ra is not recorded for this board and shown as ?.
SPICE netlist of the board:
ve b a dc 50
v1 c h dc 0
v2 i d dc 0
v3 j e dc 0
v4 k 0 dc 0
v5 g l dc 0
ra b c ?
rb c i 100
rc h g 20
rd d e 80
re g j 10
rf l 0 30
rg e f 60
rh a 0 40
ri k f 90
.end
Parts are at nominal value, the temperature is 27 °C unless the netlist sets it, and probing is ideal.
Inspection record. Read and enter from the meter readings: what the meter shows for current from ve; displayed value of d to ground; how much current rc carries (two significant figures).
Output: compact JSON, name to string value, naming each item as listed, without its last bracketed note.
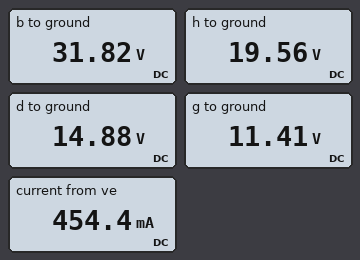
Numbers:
{"what the meter shows for current from ve": "454.4 mA", "displayed value of d to ground": "14.88 V", "how much current rc carries": "410 mA"}
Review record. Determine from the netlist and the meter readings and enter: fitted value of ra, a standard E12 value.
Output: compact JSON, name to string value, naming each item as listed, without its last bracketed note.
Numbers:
{"fitted value of ra, a standard E12 value": "27 Ω"}
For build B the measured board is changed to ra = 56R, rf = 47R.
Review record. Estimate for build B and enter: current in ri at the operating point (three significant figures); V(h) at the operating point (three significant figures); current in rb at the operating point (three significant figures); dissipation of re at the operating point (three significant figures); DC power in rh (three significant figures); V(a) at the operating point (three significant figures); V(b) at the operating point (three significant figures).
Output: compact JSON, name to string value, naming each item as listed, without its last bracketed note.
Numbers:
{"current in ri at the operating point": "77.4 mA", "V(h) at the operating point": "18.0 V", "current in rb at the operating point": "35.4 mA", "dissipation of re at the operating point": "17.6 mW", "DC power in rh": "4.45 W", "V(a) at the operating point": "-13.3 V", "V(b) at the operating point": "36.7 V"}
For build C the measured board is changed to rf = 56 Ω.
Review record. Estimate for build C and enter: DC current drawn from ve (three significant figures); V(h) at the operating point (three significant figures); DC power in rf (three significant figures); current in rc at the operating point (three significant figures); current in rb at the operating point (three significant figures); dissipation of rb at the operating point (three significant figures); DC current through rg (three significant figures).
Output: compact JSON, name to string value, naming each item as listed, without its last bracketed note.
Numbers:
{"DC current drawn from ve": "397 mA", "V(h) at the operating point": "23.4 V", "DC power in rf": "4.77 W", "current in rc at the operating point": "354 mA", "current in rb at the operating point": "42.8 mA", "dissipation of rb at the operating point": "183 mW", "DC current through rg": "105 mA"}
